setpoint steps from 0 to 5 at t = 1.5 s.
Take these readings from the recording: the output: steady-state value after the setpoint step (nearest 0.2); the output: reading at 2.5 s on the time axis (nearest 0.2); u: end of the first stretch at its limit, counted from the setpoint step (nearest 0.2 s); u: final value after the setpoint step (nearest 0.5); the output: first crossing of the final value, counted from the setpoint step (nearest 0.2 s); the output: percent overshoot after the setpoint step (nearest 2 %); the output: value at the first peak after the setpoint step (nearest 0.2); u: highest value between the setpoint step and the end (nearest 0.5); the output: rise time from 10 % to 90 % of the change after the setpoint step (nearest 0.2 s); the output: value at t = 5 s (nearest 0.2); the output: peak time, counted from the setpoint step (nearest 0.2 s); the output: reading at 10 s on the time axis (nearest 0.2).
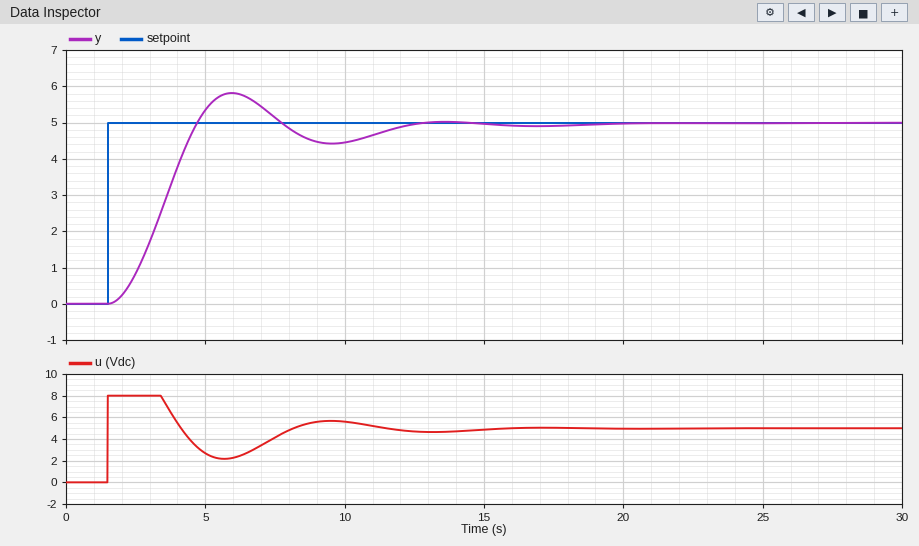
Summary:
5.0
0.8
2.0 s
5.0
3.2 s
16 %
5.8
8.0
2.2 s
5.4
4.4 s
4.4
